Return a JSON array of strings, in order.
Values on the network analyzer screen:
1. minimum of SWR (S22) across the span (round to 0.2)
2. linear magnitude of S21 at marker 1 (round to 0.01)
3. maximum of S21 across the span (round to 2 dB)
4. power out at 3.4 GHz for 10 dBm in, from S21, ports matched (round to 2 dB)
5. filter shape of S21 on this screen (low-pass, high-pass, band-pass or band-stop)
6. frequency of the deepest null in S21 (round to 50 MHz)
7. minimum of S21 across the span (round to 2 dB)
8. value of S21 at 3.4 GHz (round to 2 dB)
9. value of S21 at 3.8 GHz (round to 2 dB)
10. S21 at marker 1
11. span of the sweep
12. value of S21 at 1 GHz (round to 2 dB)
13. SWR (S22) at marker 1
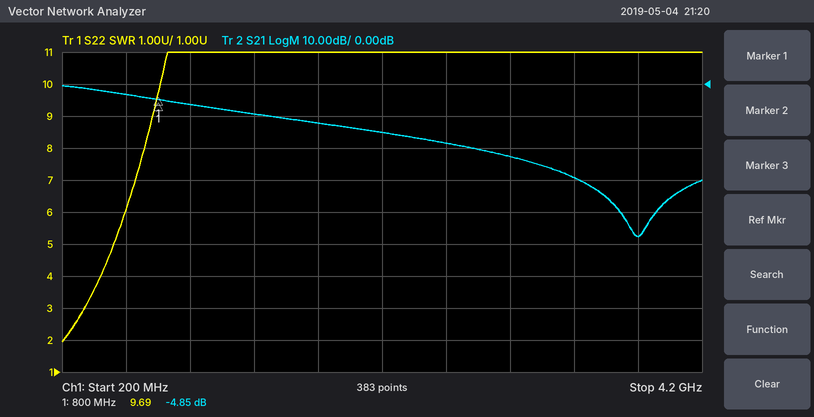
["2.0", "0.57", "0 dB", "-20 dBm", "low-pass", "3.80 GHz", "-48 dB", "-30 dB", "-48 dB", "-4.85 dB", "4 GHz", "-6 dB", "9.69"]
